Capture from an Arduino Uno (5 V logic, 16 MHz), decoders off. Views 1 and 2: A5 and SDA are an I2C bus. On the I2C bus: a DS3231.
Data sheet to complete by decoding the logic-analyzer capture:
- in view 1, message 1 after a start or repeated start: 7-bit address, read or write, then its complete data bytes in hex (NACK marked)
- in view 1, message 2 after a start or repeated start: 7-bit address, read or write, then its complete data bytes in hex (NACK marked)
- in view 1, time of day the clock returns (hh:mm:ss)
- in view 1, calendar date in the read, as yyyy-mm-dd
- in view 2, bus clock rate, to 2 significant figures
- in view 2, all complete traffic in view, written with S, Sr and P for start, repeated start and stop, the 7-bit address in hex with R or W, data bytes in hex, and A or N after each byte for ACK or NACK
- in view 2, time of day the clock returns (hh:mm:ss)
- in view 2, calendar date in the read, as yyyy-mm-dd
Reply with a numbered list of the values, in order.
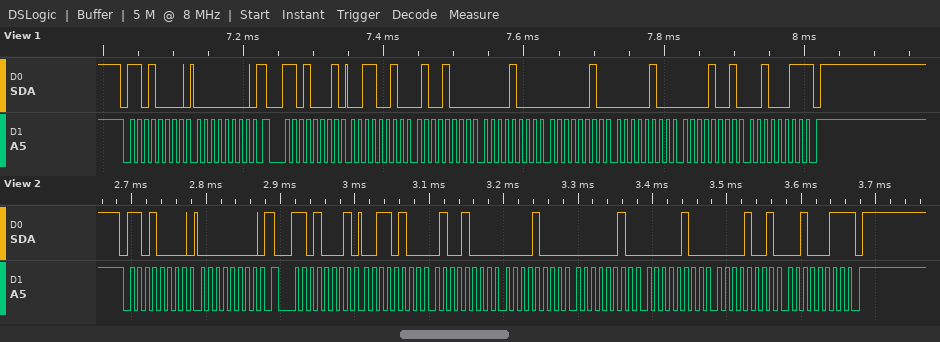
1. 0x68 write: 00
2. 0x68 read: 32 48 08 02 04 09 23 NACK
3. 08:48:32
4. 2023-09-04
5. 100 kHz
6. S 68W A 00 A Sr 68R A 34 A 48 A 08 A 02 A 04 A 09 A 23 N P
7. 08:48:34
8. 2023-09-04
